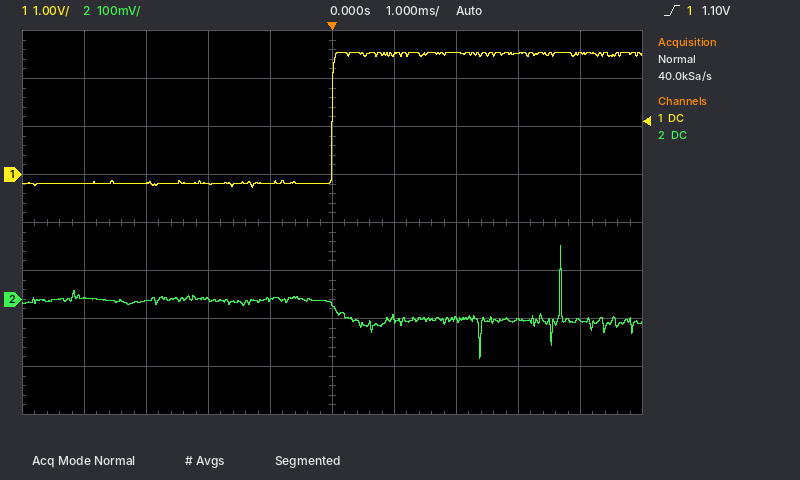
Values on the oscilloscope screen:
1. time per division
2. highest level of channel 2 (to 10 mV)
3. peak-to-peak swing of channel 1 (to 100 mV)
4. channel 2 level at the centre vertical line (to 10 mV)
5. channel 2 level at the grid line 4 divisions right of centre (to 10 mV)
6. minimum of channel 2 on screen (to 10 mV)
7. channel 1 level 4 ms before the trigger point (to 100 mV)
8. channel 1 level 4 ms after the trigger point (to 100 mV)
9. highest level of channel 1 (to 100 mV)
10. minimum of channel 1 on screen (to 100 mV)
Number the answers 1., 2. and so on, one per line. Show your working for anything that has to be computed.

1. 1 ms
2. 110 mV
3. 2.5 V − (-300 mV) = 2.8 V
4. -10 mV
5. -40 mV
6. -120 mV
7. -200 mV
8. 2.5 V
9. 2.5 V
10. -300 mV
